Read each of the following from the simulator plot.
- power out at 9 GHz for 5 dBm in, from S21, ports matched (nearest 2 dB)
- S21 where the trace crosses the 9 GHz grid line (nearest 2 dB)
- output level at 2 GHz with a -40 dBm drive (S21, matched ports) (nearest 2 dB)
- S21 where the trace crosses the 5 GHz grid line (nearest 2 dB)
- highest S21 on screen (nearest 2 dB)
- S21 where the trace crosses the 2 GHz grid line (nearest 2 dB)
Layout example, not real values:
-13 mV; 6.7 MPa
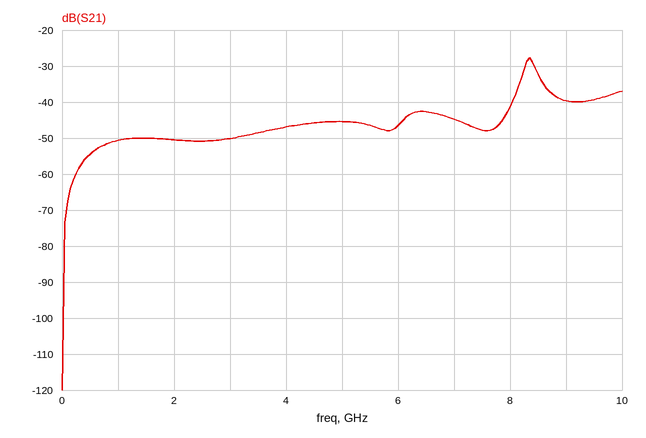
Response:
-34 dBm; -40 dB; -90 dBm; -46 dB; -28 dB; -50 dB
